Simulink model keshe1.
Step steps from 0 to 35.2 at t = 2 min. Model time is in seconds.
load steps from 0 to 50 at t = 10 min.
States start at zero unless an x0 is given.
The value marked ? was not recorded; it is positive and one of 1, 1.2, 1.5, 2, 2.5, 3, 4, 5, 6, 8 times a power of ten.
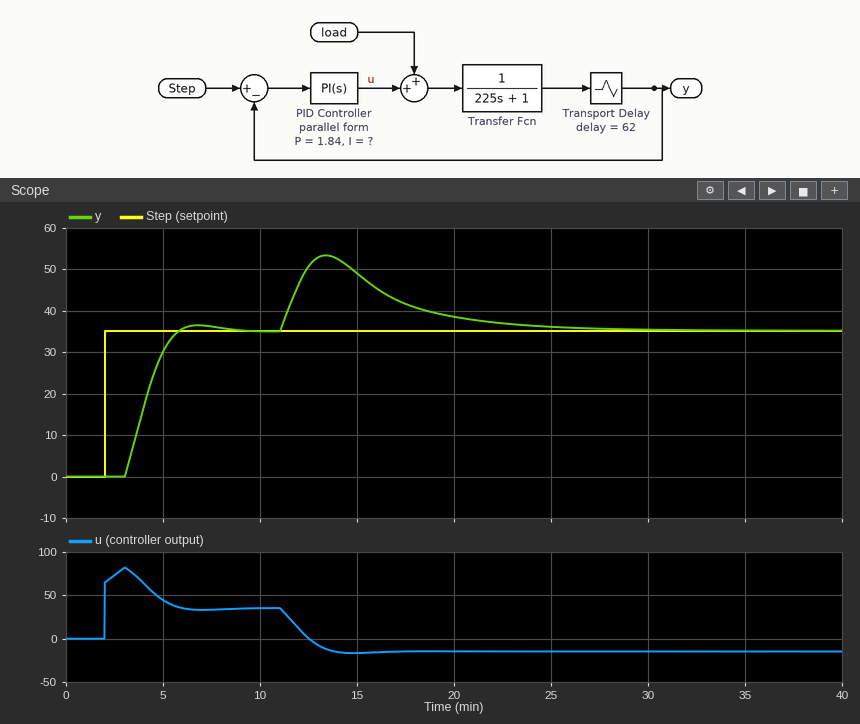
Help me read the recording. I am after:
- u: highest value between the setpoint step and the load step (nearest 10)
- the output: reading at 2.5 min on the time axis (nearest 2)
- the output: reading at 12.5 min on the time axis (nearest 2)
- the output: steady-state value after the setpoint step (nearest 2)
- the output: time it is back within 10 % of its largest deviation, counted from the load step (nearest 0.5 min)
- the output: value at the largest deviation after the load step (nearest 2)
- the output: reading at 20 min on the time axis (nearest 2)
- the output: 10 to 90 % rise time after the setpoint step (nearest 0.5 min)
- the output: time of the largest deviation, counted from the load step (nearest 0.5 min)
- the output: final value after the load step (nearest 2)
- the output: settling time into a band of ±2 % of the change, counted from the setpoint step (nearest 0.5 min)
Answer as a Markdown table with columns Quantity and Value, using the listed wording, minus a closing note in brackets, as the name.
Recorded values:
| Quantity | Value |
|---|---|
| u: highest value between the setpoint step and the load step | 80 |
| the output: reading at 2.5 min on the time axis | 0 |
| the output: reading at 12.5 min on the time axis | 50 |
| the output: steady-state value after the setpoint step | 36 |
| the output: time it is back within 10 % of its largest deviation, counted from the load step | 12.5 min |
| the output: value at the largest deviation after the load step | 54 |
| the output: reading at 20 min on the time axis | 38 |
| the output: 10 to 90 % rise time after the setpoint step | 2.0 min |
| the output: time of the largest deviation, counted from the load step | 3.5 min |
| the output: final value after the load step | 36 |
| the output: settling time into a band of ±2 % of the change, counted from the setpoint step | 6.0 min |
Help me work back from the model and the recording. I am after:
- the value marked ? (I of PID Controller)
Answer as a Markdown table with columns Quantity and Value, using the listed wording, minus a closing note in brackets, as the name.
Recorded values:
| Quantity | Value |
|---|---|
| the value marked ? | 0.008 |
